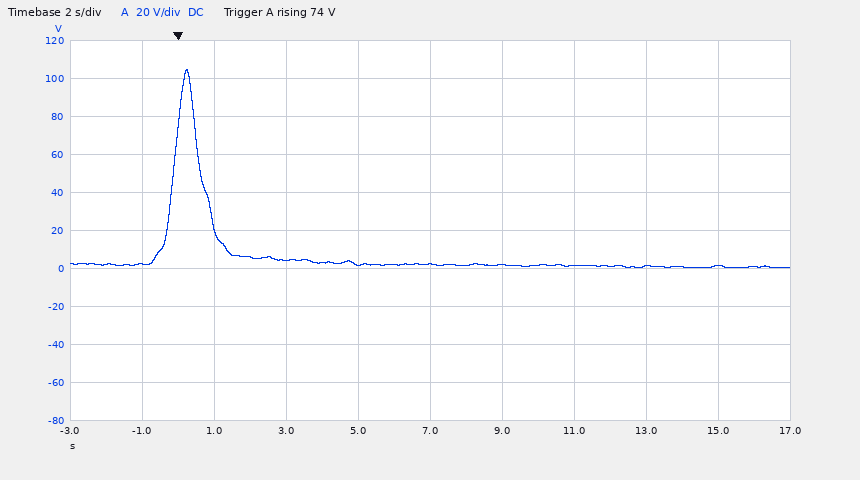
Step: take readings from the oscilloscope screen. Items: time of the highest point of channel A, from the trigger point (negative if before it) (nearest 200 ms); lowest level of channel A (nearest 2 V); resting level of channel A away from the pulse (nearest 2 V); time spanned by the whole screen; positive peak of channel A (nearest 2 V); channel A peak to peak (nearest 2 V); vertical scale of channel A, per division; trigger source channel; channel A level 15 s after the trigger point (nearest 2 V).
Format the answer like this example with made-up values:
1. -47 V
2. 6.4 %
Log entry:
1. +200 ms
2. 0 V
3. 2 V
4. 20 s
5. 104 V
6. 104 V
7. 20 V
8. channel A
9. 2 V
